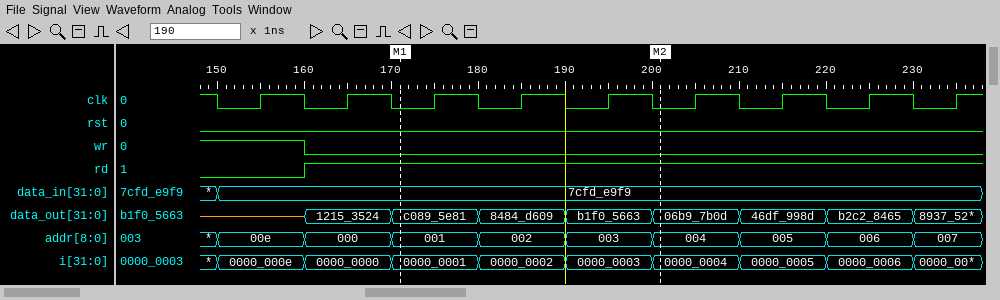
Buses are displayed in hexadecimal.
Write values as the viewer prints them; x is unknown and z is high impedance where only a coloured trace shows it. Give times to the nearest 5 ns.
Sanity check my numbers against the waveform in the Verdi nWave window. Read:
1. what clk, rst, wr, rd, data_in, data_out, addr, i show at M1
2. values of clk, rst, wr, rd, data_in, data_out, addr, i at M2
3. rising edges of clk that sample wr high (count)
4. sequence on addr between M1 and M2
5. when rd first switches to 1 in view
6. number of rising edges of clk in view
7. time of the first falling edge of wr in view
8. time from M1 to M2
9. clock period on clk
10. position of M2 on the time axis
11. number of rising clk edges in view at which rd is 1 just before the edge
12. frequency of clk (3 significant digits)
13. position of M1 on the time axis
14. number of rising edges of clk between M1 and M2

clk=0, rst=0, wr=0, rd=1, data_in=7cfd_e9f9, data_out=c089_5e81, addr=001, i=0000_0001
clk=0, rst=0, wr=0, rd=1, data_in=7cfd_e9f9, data_out=06b9_7b0d, addr=004, i=0000_0004
1
001, 002, 003, 004
160 ns
9
160 ns
30 ns
10 ns
200 ns
8
100 MHz
170 ns
3
